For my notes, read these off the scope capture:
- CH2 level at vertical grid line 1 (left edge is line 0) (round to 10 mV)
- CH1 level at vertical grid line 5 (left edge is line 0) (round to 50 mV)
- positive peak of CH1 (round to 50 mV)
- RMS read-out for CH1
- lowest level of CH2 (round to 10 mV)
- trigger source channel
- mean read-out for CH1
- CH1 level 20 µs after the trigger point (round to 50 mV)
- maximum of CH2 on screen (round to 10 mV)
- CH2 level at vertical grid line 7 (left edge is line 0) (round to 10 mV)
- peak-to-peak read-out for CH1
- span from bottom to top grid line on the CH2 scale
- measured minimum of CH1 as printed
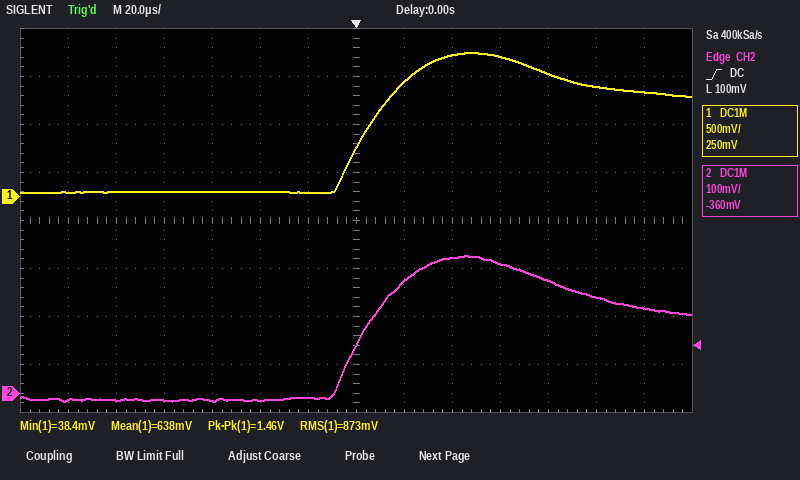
-10 mV
50 mV
1.50 V
873 mV
-20 mV
CH2
638 mV
1.20 V
290 mV
100 mV
1.46 V
800 mV
38.4 mV
